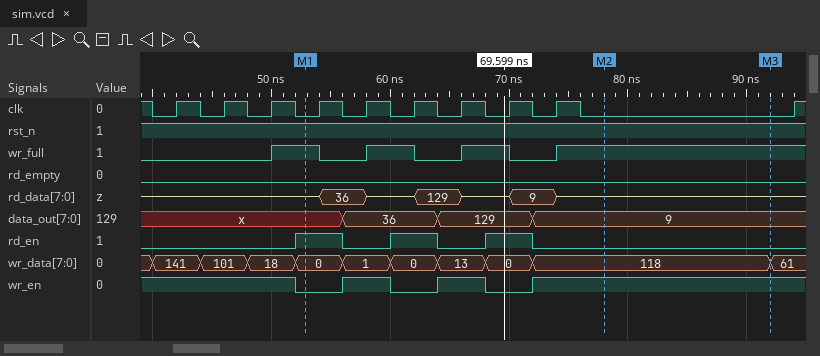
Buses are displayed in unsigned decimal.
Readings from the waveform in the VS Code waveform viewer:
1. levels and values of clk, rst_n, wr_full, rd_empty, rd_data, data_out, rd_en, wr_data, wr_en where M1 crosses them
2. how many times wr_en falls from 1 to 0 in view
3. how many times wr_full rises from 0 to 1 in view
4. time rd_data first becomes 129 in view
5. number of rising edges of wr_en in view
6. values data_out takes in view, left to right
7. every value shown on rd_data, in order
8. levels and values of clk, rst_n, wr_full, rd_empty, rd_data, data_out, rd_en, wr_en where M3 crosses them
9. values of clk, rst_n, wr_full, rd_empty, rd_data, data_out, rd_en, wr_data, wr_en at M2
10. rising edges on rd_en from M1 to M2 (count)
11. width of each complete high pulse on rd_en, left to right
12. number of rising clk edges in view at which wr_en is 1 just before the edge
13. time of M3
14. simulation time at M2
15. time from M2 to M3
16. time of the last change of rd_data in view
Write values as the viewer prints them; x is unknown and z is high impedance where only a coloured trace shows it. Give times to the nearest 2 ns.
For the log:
clk=0, rst_n=1, wr_full=1, rd_empty=0, rd_data=z, data_out=x, rd_en=1, wr_data=0, wr_en=0
3
4
62 ns
3
x, 36, 129, 9
z, 36, z, 129, z, 9, z
clk=0, rst_n=1, wr_full=1, rd_empty=0, rd_data=z, data_out=9, rd_en=0, wr_en=1
clk=0, rst_n=1, wr_full=1, rd_empty=0, rd_data=z, data_out=9, rd_en=0, wr_data=118, wr_en=1
2
4 ns, 4 ns, 4 ns
7
92 ns
78 ns
14 ns
74 ns
